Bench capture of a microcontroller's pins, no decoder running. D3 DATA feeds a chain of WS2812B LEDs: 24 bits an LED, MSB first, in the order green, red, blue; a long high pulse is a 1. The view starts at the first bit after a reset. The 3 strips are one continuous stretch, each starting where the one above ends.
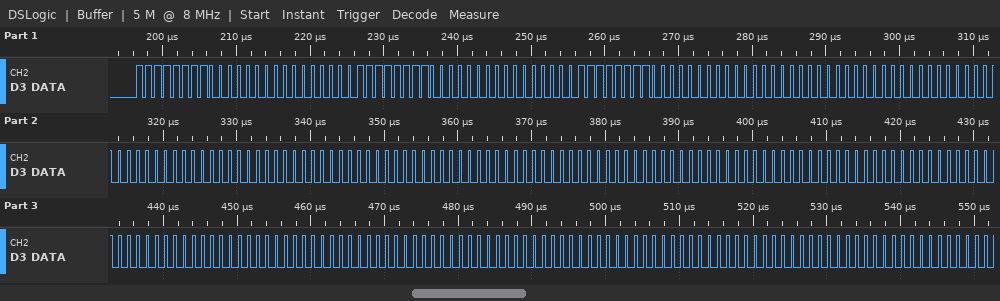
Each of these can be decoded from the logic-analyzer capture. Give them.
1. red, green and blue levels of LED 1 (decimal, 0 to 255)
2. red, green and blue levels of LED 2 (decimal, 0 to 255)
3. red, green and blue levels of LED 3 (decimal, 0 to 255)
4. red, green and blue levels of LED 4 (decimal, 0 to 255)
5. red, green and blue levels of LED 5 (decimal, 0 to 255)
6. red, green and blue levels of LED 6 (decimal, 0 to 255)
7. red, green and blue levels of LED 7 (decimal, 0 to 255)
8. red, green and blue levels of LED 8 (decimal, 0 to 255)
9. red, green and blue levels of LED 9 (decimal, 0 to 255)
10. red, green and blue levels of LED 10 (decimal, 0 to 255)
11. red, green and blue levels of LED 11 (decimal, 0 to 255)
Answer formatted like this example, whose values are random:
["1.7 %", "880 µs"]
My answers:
["0, 255, 0", "0, 255, 0", "0, 255, 0", "0, 0, 0", "0, 0, 0", "0, 0, 0", "0, 0, 0", "0, 0, 0", "0, 0, 0", "0, 0, 0", "0, 0, 0"]
